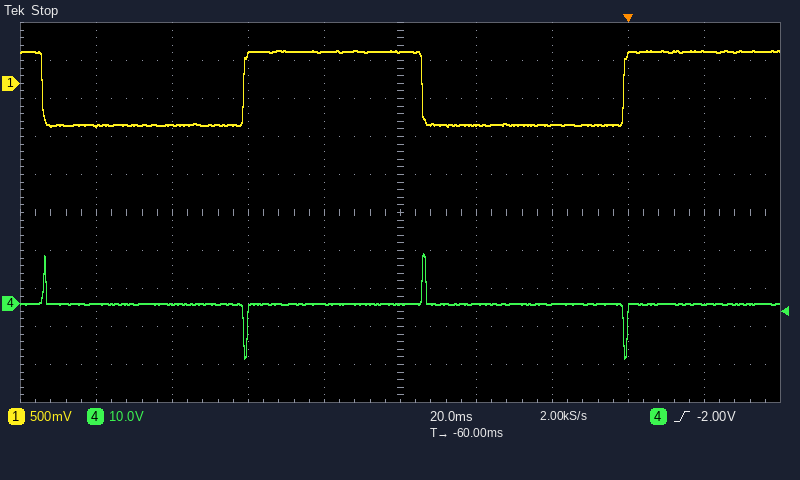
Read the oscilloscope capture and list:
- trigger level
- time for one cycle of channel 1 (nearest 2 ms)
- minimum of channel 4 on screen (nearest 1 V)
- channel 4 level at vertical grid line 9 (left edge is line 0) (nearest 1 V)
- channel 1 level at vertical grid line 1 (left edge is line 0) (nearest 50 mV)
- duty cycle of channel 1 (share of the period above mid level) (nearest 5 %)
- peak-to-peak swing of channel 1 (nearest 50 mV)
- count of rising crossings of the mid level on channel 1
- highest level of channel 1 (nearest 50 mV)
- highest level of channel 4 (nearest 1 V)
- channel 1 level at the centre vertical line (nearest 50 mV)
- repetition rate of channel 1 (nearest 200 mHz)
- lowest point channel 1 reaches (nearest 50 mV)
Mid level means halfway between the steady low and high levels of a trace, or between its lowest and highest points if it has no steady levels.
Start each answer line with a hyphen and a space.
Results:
- -2.00 V
- 100 ms
- -14 V
- 0 V
- -550 mV
- 45 %
- 1.00 V
- 2
- 450 mV
- 13 V
- 400 mV
- 10.0 Hz
- -550 mV
